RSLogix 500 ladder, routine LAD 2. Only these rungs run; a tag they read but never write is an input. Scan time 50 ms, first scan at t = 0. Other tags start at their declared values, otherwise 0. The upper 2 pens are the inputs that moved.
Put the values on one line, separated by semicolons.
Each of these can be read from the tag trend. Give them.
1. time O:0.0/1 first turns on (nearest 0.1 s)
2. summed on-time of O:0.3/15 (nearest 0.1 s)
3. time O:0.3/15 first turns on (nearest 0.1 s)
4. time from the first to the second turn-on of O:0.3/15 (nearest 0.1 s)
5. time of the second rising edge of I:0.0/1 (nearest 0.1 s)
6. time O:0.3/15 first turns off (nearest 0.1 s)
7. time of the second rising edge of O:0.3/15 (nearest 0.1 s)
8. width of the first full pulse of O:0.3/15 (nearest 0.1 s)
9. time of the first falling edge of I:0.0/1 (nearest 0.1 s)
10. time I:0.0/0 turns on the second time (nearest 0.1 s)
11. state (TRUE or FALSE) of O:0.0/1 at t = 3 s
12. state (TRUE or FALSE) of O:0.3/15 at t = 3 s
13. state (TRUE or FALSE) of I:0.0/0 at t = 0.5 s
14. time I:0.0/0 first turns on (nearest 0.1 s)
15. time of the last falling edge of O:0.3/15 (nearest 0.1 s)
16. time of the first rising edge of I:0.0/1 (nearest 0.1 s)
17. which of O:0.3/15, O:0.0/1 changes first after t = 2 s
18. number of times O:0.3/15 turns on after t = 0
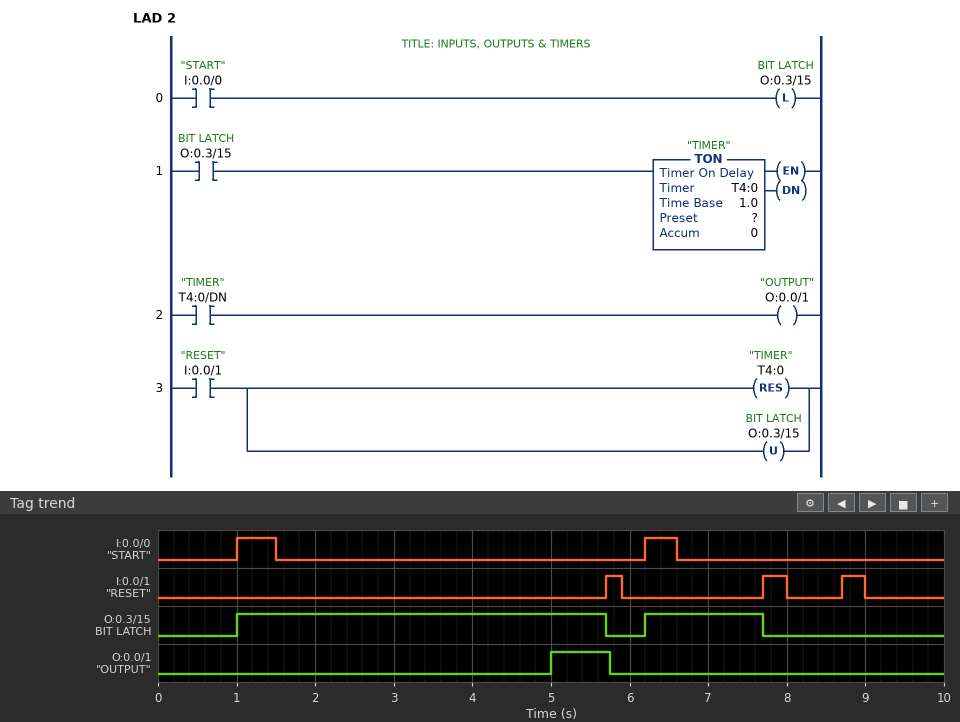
5.0 s; 6.2 s; 1.0 s; 5.2 s; 7.7 s; 5.7 s; 6.2 s; 4.7 s; 5.9 s; 6.2 s; FALSE; TRUE; FALSE; 1.0 s; 7.7 s; 5.7 s; O:0.0/1; 2
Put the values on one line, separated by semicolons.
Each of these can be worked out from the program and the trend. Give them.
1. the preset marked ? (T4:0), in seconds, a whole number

4 s
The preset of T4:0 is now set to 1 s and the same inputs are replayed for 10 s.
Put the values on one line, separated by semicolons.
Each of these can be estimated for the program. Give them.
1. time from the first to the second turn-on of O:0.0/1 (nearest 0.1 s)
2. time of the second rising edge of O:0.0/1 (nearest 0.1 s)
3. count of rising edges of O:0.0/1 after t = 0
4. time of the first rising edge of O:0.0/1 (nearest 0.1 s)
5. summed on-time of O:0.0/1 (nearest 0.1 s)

5.2 s; 7.2 s; 2; 2.0 s; 4.3 s
